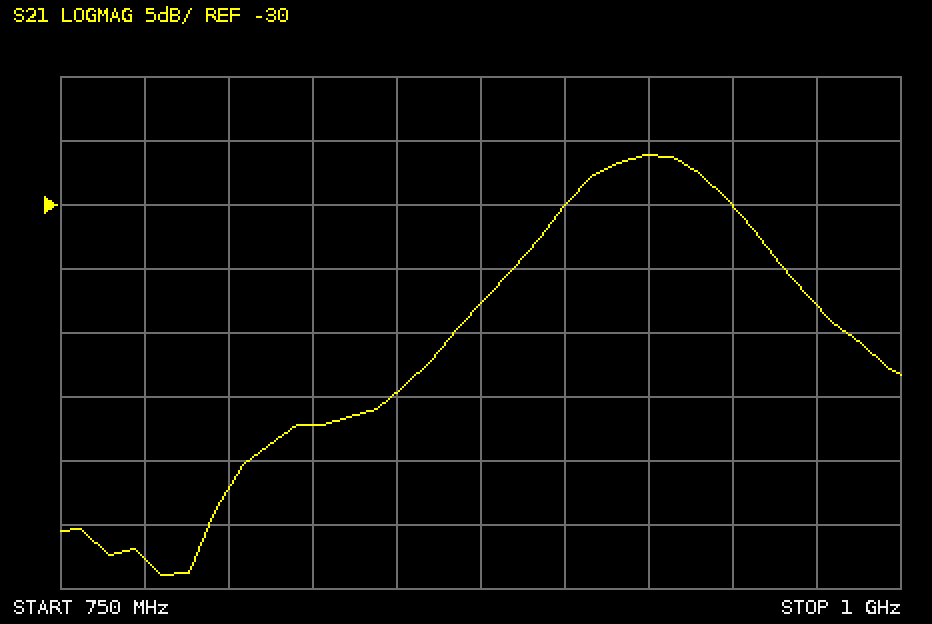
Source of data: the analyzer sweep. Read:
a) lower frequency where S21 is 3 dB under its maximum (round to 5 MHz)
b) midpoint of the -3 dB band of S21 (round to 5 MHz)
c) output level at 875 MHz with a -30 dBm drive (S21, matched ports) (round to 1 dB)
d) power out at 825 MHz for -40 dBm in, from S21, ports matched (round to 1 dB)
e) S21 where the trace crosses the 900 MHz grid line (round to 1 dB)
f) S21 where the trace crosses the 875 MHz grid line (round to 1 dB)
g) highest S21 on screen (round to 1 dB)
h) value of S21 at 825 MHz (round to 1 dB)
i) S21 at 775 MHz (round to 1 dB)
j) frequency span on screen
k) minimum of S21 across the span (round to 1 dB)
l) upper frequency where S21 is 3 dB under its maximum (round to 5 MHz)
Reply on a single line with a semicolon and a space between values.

905 MHz; 925 MHz; -68 dBm; -87 dBm; -30 dB; -38 dB; -26 dB; -47 dB; -58 dB; 250 MHz; -59 dB; 945 MHz
